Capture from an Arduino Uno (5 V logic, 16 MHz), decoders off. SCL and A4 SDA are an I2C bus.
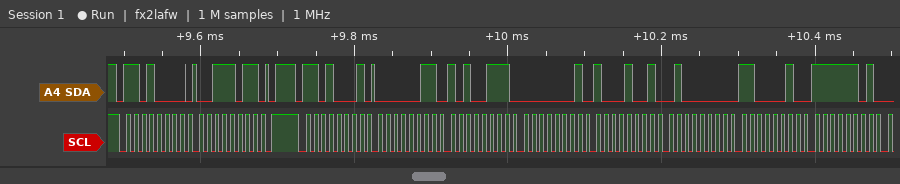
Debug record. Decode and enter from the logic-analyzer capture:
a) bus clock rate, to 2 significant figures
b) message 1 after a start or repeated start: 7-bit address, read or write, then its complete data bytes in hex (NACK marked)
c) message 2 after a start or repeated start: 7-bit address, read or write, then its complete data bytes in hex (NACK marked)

100 kHz
0x68 write: 3B
0x68 read: 03 A7 01 89 40 C2 FD
